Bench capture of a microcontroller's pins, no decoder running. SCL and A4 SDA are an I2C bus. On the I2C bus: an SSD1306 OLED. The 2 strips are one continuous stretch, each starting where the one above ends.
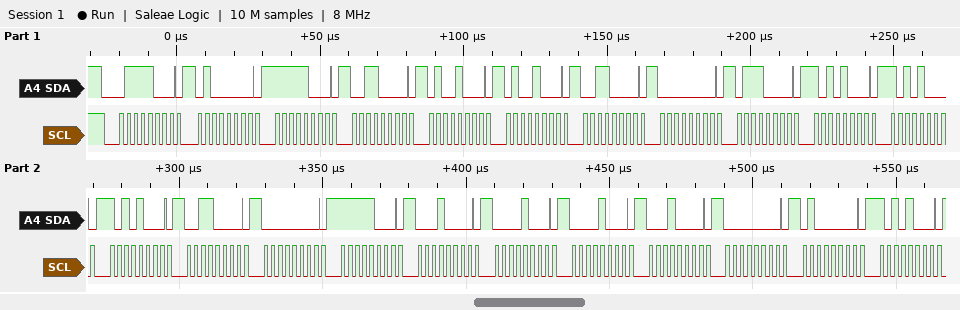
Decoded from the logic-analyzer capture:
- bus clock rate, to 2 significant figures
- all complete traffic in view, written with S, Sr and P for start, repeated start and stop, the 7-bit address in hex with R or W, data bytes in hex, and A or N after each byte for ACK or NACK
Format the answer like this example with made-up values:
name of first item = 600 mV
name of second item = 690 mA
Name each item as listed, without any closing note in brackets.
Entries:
bus clock rate, to 2 significant figures = 400 kHz
all complete traffic in view, written with S, Sr and P for start, repeated start and stop, the 7-bit address in hex with R or W, data bytes in hex, and A or N after each byte for ACK or NACK = S 3CW A 40 A F8 A 30 A 48 A 48 A 30 A 00 A 70 A A8 A A8 A A8 A 30 A 00 A F8 A 10 A 08 A 08 A 10 A 00 A 40 A A8 A
